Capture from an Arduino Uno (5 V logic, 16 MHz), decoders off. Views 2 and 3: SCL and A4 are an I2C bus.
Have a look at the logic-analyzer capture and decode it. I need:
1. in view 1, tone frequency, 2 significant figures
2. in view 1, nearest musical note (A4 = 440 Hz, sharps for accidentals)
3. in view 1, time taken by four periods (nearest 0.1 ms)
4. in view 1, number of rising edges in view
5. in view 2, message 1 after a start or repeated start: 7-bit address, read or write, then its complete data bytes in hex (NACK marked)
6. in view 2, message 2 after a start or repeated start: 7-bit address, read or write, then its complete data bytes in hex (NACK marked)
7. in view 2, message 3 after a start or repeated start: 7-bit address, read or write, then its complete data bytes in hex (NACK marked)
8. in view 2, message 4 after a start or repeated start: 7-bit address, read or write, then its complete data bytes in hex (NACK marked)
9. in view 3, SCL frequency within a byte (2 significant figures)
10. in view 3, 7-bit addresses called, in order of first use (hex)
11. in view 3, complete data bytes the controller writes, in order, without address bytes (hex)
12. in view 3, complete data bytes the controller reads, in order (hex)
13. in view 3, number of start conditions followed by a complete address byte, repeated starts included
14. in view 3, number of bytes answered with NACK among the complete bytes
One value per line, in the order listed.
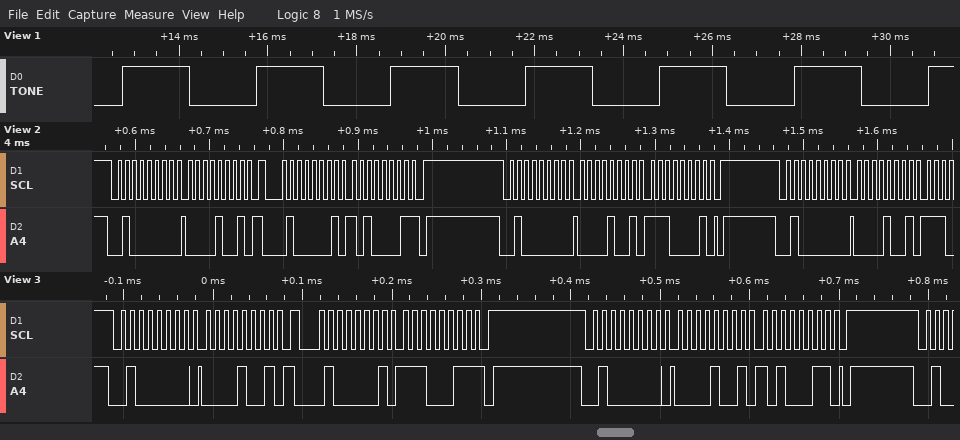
330 Hz
E4
12.1 ms
7
0x20 write: 09
0x20 read: A1 NACK
0x20 write: 09 E1
0x20 write: 09
100 kHz
0x20
09 09 A3
E3
3
1
